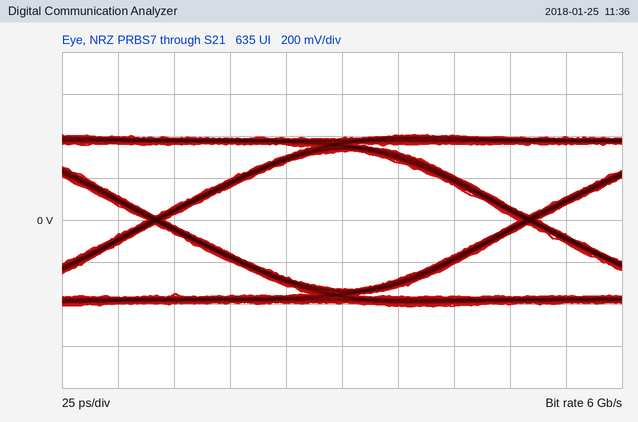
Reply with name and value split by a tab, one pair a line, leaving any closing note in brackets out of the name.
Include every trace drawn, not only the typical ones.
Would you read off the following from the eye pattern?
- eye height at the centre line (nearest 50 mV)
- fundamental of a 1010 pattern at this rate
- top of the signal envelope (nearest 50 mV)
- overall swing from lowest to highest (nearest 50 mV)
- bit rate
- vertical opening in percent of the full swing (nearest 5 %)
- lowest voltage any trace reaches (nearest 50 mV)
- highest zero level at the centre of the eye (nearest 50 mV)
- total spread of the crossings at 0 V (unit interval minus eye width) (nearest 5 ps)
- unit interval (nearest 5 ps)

eye height at the centre line	650 mV
fundamental of a 1010 pattern at this rate	3 GHz
top of the signal envelope	400 mV
overall swing from lowest to highest	800 mV
bit rate	6 Gb/s
vertical opening in percent of the full swing	80 %
lowest voltage any trace reaches	-400 mV
highest zero level at the centre of the eye	-350 mV
total spread of the crossings at 0 V (unit interval minus eye width)	10 ps
unit interval	165 ps
